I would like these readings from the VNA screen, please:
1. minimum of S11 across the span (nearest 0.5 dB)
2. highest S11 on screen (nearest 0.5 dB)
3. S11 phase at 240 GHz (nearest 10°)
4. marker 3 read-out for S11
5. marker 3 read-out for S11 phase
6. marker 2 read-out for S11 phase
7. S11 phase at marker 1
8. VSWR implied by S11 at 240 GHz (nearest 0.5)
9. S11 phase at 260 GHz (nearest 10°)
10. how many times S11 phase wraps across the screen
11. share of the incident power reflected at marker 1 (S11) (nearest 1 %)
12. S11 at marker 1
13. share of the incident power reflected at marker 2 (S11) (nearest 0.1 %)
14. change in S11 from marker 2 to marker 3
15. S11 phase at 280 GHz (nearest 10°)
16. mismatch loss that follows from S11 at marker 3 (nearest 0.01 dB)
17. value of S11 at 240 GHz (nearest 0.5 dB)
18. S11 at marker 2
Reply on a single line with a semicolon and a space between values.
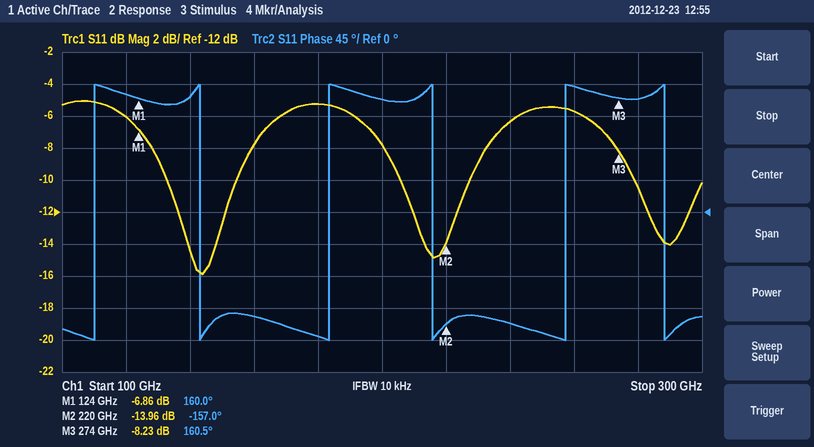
-16.0 dB; -5.0 dB; -160°; -8.23 dB; 160.5°; -157.0°; 160.0°; 3.0; 180°; 6; 21 %; -6.86 dB; 4.0 %; 5.73 dB; 160°; 0.71 dB; -6.5 dB; -13.96 dB
